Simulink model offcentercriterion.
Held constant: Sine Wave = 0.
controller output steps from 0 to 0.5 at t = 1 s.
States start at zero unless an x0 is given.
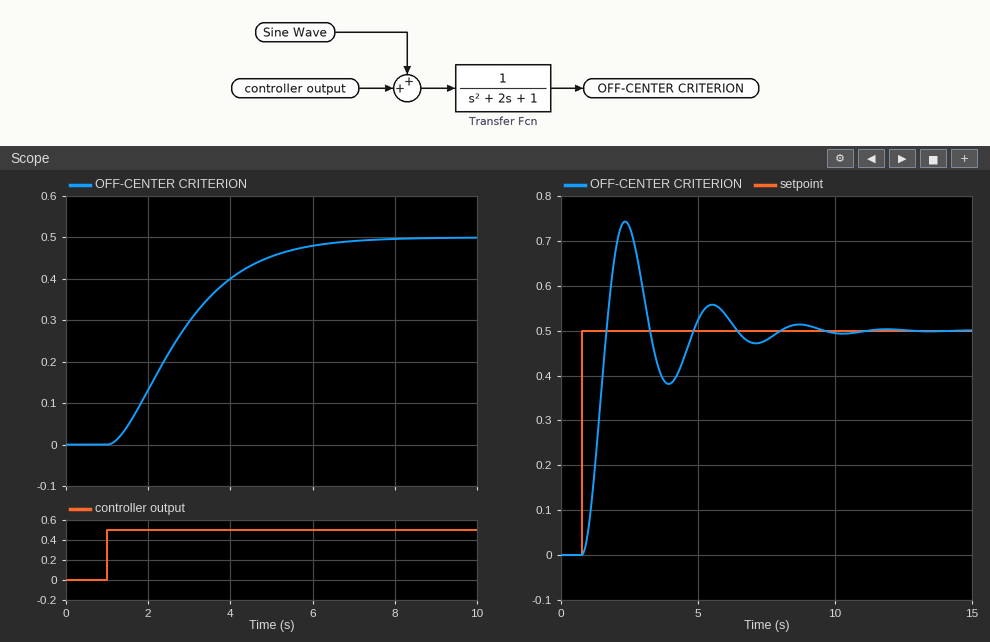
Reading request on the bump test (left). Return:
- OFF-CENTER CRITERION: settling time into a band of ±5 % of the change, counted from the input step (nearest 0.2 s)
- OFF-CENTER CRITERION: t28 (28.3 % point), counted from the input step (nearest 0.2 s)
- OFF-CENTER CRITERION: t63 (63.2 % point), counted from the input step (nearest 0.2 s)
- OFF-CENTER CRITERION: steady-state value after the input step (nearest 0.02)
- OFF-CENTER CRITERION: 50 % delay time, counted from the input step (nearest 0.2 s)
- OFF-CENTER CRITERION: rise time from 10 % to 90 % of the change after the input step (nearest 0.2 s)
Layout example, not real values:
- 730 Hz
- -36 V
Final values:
- 4.8 s
- 1.0 s
- 2.2 s
- 0.50
- 1.6 s
- 3.4 s
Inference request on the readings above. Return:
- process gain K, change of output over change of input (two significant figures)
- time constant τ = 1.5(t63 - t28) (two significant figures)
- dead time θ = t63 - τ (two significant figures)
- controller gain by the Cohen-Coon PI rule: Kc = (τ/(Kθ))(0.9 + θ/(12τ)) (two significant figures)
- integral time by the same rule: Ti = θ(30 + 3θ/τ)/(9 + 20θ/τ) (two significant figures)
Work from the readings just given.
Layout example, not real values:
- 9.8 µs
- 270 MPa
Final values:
- 1.0
- 1.8 s
- 0.40 s
- 4.1
- 0.91 s
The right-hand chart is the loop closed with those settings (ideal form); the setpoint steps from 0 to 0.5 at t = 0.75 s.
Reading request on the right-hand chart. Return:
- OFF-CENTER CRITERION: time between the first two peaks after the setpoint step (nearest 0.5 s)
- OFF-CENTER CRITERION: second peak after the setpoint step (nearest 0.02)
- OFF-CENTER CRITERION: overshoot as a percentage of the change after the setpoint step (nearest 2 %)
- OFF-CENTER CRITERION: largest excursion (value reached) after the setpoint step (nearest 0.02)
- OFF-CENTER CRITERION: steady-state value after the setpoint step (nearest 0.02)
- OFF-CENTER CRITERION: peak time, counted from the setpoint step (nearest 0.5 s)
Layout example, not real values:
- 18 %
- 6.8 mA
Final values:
- 3.0 s
- 0.56
- 48 %
- 0.74
- 0.50
- 1.5 s
